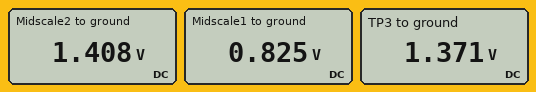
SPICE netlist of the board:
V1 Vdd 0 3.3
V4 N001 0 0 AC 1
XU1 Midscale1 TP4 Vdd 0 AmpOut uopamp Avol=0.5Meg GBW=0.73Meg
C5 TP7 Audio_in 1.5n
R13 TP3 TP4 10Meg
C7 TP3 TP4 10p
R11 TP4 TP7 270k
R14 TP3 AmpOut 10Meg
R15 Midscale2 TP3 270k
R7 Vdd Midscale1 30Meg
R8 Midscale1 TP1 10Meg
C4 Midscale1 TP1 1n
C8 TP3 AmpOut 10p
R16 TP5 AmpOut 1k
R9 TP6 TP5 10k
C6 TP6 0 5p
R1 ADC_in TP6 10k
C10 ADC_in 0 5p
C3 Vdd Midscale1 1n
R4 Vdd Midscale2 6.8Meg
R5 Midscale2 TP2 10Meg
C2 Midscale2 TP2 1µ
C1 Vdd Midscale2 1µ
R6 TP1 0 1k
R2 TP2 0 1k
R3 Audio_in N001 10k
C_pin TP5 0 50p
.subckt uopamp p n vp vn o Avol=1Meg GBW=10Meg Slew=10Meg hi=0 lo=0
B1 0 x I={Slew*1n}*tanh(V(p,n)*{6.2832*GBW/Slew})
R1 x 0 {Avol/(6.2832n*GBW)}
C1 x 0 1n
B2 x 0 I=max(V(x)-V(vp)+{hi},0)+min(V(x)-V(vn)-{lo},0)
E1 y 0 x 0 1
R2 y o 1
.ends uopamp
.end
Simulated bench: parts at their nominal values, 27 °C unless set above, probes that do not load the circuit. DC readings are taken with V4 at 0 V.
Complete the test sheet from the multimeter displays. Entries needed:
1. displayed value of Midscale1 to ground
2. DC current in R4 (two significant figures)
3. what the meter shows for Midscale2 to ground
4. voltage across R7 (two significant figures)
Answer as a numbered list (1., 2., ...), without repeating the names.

1. 0.825 V
2. 280 nA
3. 1.408 V
4. 2.5 V
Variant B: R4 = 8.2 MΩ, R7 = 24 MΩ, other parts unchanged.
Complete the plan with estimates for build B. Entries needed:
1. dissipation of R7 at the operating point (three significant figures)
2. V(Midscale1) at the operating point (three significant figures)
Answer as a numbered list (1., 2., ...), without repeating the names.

1. 226 nW
2. 971 mV
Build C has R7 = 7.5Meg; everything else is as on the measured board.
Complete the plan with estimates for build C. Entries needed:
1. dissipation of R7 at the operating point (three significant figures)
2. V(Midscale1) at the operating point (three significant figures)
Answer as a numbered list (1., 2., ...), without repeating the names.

1. 267 nW
2. 1.89 V
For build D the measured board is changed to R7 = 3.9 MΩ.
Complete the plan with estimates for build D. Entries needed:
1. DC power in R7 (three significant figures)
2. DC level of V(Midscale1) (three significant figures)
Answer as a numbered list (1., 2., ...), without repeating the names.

1. 220 nW
2. 2.37 V
